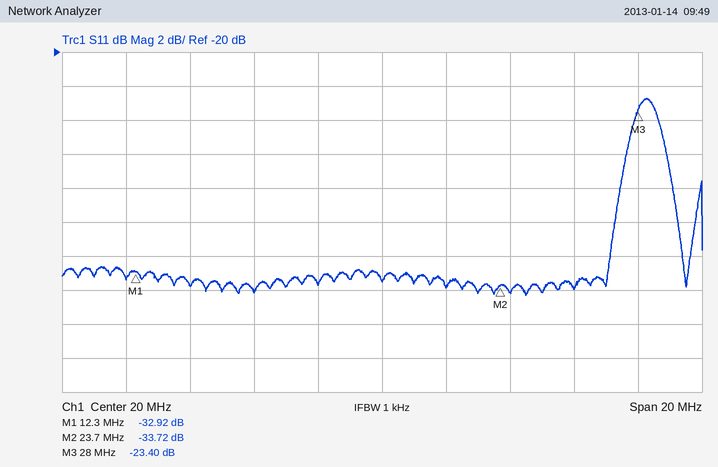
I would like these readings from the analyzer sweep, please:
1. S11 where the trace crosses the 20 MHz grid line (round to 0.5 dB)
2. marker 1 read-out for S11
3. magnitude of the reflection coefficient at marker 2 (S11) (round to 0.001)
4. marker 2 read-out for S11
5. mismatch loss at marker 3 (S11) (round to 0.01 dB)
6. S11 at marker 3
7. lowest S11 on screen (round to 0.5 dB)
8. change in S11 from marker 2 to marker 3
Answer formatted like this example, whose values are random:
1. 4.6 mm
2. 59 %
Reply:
1. -33.5 dB
2. -32.92 dB
3. 0.021
4. -33.72 dB
5. 0.02 dB
6. -23.40 dB
7. -34.5 dB
8. 10.32 dB
